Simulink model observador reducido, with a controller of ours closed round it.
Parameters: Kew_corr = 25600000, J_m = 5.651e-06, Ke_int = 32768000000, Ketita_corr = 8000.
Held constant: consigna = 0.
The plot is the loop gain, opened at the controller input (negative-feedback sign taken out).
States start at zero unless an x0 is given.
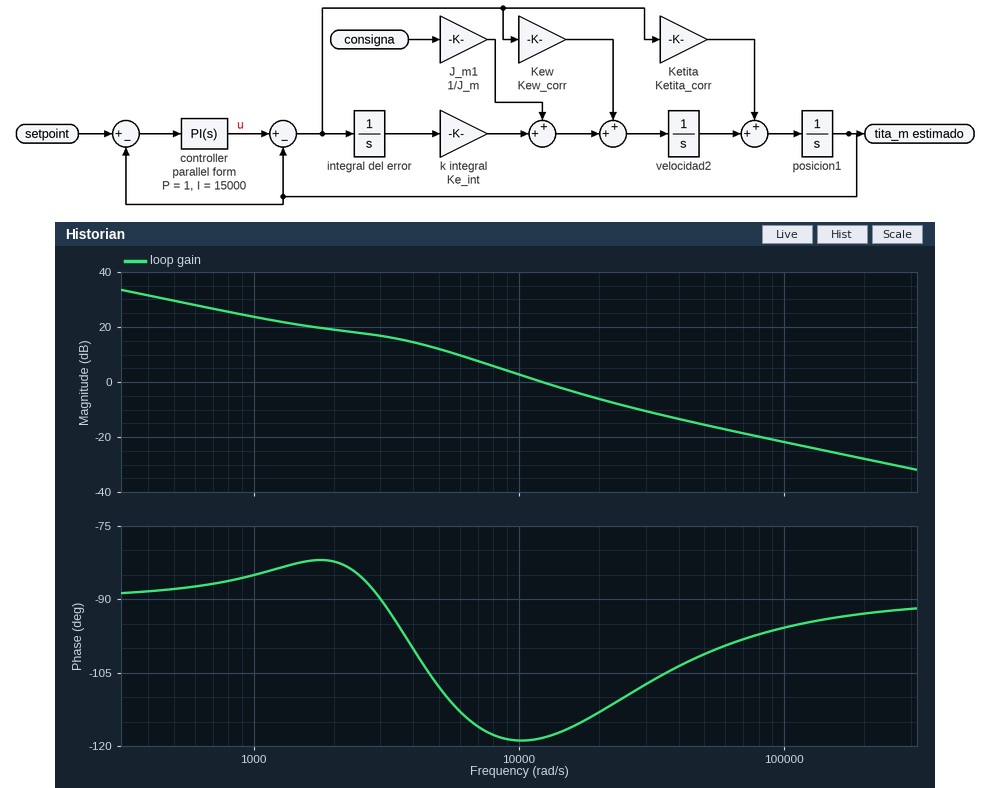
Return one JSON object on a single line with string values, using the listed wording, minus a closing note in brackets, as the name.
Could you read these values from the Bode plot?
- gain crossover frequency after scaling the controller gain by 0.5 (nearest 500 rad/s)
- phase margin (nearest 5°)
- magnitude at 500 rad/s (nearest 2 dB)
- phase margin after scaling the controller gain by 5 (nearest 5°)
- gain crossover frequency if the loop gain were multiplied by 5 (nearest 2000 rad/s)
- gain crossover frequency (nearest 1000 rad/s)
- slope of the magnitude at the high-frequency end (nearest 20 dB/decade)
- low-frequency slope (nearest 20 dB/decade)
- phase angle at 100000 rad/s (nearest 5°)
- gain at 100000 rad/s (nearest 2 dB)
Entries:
{"gain crossover frequency after scaling the controller gain by 0.5": "8000 rad/s", "phase margin": "60°", "magnitude at 500 rad/s": "30 dB", "phase margin after scaling the controller gain by 5": "75°", "gain crossover frequency if the loop gain were multiplied by 5": "42000 rad/s", "gain crossover frequency": "12000 rad/s", "slope of the magnitude at the high-frequency end": "-20 dB/decade", "low-frequency slope": "-20 dB/decade", "phase angle at 100000 rad/s": "-95°", "gain at 100000 rad/s": "-22 dB"}
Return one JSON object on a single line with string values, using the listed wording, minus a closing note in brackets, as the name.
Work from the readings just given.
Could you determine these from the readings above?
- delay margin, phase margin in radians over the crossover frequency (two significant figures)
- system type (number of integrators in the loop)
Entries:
{"delay margin, phase margin in radians over the crossover frequency": "0.000087 s", "system type": "1"}
